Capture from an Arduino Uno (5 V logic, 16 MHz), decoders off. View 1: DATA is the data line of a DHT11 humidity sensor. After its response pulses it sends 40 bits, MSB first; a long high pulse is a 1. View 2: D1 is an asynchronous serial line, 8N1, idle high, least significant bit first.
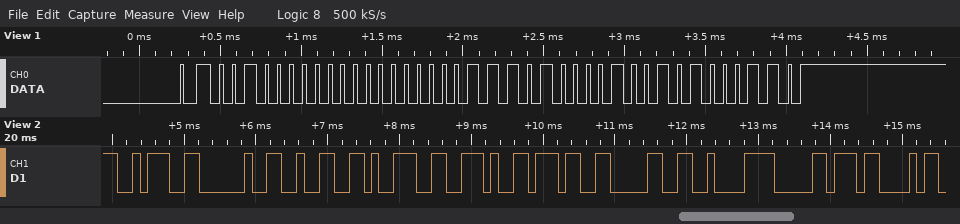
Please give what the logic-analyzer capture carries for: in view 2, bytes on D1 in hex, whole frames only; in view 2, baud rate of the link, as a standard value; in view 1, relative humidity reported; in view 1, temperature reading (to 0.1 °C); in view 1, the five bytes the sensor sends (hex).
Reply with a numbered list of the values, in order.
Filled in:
1. 3A 20 32 39 2E 37 30 C2 B0 43
2. 9600 baud
3. 32 %
4. 29.9 °C
5. 20 00 1D 09 46
